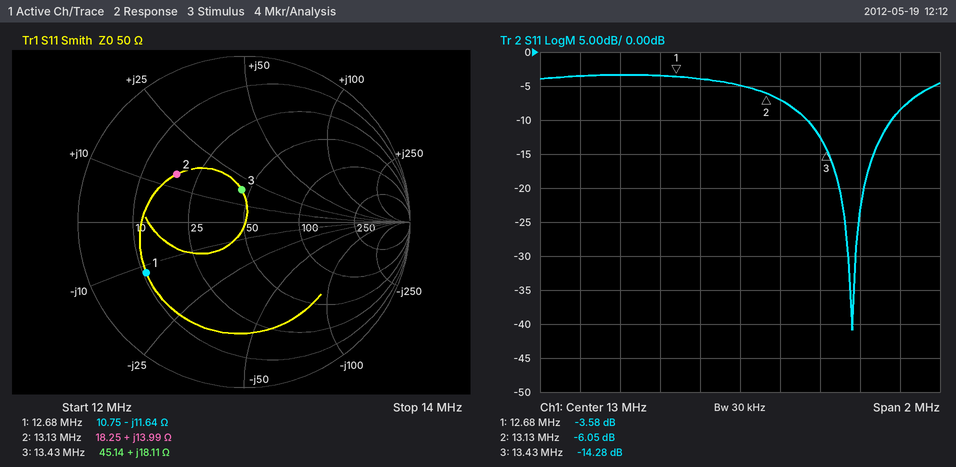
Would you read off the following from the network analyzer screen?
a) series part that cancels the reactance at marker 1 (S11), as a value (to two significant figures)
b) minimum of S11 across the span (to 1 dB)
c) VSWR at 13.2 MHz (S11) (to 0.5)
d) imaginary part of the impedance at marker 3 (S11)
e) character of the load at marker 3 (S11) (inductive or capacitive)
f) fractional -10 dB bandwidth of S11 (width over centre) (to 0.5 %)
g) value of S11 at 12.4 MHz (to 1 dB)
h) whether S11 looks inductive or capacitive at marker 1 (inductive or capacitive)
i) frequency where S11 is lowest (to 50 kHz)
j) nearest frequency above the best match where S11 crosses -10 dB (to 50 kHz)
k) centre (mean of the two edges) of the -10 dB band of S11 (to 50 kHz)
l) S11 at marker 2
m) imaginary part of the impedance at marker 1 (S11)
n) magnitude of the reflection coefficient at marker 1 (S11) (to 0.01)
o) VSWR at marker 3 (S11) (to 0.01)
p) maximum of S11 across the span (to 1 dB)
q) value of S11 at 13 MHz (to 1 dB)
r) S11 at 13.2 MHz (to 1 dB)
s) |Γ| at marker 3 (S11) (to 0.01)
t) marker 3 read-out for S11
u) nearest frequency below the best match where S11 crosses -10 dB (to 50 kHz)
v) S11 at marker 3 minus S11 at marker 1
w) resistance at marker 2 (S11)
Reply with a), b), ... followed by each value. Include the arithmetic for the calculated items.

a) L = 11.64 Ω/(2π × 12.68 MHz) ≈ 146 nH, so 150 nH to two significant figures
b) -41 dB
c) |Γ| = 10^(-7/20) = 0.4467; VSWR = (1 + 0.4467)/(1 − 0.4467) ≈ 2.61, so 2.5 to the nearest 0.5
d) +18.11 Ω
e) inductive
f) 400 kHz / 13.55 MHz ≈ 3.0 %
g) -3 dB
h) capacitive
i) 13.55 MHz
j) 13.75 MHz
k) 13.55 MHz
l) -6.05 dB
m) -11.64 Ω
n) 0.66
o) (1 + 0.1932)/(1 − 0.1932) ≈ 1.48
p) -3 dB
q) -5 dB
r) -7 dB
s) 0.19
t) -14.28 dB
u) 13.35 MHz
v) -14.28 − (-3.58) = -10.70 dB
w) 18.25 Ω
